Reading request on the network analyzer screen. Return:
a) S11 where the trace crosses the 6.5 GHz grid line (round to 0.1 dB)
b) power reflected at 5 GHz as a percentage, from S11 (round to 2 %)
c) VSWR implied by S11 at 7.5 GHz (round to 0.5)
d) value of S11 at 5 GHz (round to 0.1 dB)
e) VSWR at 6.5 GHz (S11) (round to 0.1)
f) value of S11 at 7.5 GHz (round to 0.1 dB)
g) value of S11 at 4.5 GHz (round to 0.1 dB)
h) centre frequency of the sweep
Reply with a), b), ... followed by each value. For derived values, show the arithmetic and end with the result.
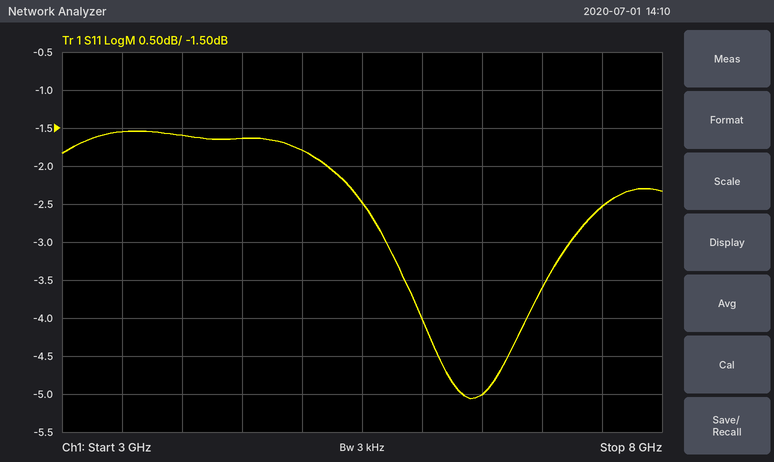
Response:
a) -5.0 dB
b) 10^(-1.8/10) ≈ 66 %
c) |Γ| = 10^(-2.5/20) = 0.7499; VSWR = (1 + 0.7499)/(1 − 0.7499) ≈ 7.0
d) -1.8 dB
e) |Γ| = 10^(-5/20) = 0.5623; VSWR = (1 + 0.5623)/(1 − 0.5623) ≈ 3.6
f) -2.5 dB
g) -1.6 dB
h) 5.5 GHz
